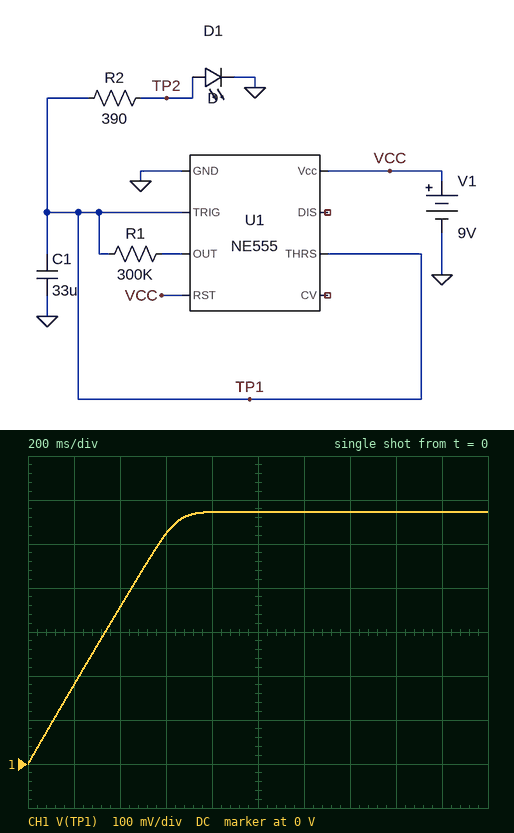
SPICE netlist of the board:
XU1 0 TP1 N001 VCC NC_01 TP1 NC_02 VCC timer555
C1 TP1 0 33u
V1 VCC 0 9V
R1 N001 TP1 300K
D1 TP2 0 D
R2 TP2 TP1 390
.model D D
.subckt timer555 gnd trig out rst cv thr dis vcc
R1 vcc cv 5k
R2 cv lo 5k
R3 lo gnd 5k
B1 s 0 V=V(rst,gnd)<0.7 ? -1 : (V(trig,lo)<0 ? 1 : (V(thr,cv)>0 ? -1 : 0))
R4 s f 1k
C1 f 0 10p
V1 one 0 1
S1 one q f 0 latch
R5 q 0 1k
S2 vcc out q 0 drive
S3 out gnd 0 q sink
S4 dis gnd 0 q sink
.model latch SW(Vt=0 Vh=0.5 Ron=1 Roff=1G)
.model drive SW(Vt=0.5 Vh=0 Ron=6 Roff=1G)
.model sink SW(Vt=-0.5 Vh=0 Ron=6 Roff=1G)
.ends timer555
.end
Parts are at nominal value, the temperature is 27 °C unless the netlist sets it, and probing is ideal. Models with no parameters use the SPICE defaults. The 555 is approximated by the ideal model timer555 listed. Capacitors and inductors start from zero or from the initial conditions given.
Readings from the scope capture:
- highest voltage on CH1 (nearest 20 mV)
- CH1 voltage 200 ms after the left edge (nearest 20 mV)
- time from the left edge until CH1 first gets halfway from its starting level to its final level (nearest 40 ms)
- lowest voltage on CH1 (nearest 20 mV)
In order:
580 mV
180 mV
320 ms
0 V
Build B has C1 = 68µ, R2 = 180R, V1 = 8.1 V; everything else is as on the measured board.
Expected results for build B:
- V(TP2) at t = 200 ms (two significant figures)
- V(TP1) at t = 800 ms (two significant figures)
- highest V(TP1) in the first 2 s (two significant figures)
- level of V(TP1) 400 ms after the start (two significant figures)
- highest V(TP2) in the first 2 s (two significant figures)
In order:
79 mV
310 mV
560 mV
160 mV
560 mV
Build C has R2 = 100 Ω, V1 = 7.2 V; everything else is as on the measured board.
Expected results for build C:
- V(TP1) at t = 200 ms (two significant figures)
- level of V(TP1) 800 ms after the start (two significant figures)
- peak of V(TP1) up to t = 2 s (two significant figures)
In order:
140 mV
540 mV
560 mV
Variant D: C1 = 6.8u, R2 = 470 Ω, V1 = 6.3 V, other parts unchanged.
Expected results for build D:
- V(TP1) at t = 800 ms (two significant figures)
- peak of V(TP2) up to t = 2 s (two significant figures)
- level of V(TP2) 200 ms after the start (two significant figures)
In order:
560 mV
550 mV
540 mV
